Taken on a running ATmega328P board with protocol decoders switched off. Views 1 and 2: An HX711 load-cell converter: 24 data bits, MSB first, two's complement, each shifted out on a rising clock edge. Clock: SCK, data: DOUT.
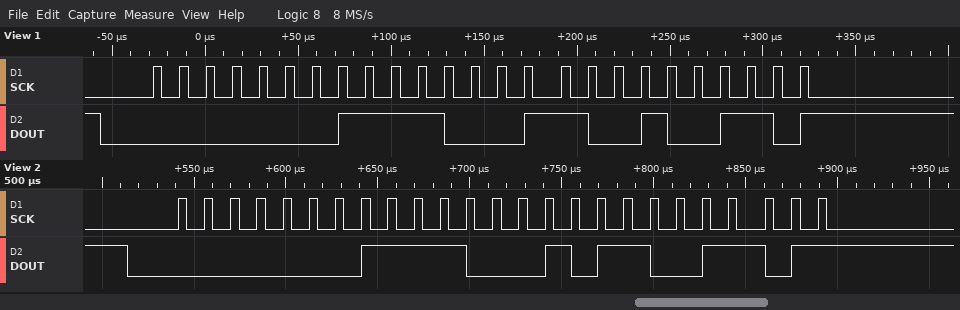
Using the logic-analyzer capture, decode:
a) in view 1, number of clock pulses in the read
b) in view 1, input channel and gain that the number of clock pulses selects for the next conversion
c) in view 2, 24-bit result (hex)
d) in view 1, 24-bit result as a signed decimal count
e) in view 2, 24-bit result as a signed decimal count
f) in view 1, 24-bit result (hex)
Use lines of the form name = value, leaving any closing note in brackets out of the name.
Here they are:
in view 1, number of clock pulses in the read = 25
in view 1, input channel and gain that the number of clock pulses selects for the next conversion = channel A, gain 128
in view 2, 24-bit result = 0x01E2CD
in view 1, 24-bit result as a signed decimal count = 123686
in view 2, 24-bit result as a signed decimal count = 123597
in view 1, 24-bit result = 0x01E326
